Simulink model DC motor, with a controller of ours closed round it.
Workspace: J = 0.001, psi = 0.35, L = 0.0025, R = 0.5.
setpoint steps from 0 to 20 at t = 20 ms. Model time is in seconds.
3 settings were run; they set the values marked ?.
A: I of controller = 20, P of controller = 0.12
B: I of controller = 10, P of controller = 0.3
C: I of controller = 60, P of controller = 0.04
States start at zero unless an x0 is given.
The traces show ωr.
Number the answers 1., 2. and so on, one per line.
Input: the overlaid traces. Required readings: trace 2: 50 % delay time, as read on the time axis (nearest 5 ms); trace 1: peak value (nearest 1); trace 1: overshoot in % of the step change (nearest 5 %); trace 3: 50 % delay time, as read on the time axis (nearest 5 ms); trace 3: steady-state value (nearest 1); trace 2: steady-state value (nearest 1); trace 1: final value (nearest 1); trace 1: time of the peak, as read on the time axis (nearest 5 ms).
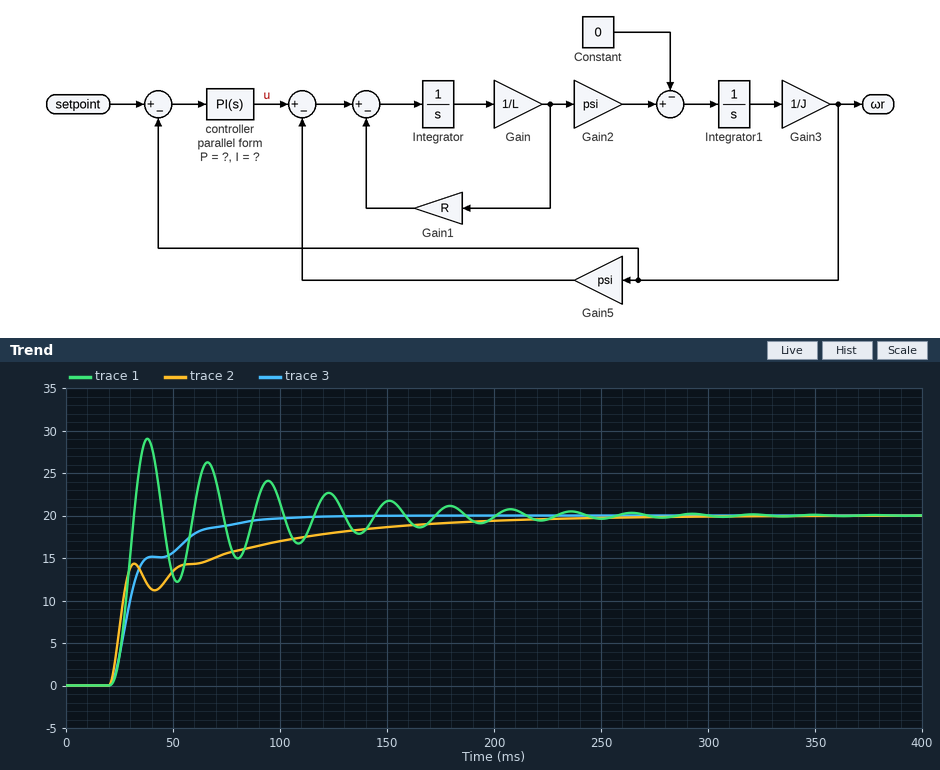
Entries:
1. 25 ms
2. 29
3. 45 %
4. 30 ms
5. 20
6. 20
7. 20
8. 40 ms
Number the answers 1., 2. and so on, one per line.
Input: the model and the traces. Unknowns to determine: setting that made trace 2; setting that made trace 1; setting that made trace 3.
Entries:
1. B
2. C
3. A
